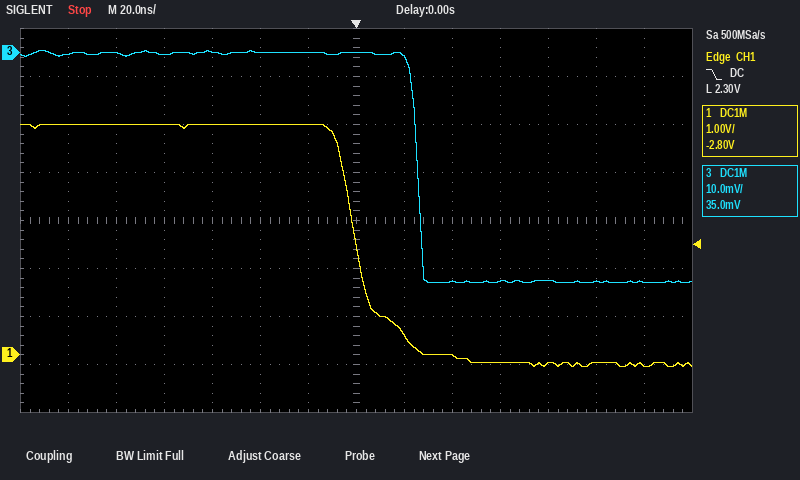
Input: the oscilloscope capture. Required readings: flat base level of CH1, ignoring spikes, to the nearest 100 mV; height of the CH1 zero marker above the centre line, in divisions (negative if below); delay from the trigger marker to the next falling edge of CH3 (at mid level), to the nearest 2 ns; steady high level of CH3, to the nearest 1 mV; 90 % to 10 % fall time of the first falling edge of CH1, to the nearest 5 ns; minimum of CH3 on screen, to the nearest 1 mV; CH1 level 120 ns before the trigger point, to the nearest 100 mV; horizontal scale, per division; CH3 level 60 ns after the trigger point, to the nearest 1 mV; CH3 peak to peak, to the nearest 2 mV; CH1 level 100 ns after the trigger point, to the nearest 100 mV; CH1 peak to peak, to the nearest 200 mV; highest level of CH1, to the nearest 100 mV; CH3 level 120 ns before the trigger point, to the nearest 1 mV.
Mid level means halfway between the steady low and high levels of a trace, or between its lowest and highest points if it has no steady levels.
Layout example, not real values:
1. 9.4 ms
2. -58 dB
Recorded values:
1. -200 mV
2. -2.8 div
3. 26 ns
4. 0 mV
5. 30 ns
6. -48 mV
7. 4.8 V
8. 20 ns
9. -48 mV
10. 48 mV
11. -200 mV
12. 5.0 V
13. 4.8 V
14. 0 mV
